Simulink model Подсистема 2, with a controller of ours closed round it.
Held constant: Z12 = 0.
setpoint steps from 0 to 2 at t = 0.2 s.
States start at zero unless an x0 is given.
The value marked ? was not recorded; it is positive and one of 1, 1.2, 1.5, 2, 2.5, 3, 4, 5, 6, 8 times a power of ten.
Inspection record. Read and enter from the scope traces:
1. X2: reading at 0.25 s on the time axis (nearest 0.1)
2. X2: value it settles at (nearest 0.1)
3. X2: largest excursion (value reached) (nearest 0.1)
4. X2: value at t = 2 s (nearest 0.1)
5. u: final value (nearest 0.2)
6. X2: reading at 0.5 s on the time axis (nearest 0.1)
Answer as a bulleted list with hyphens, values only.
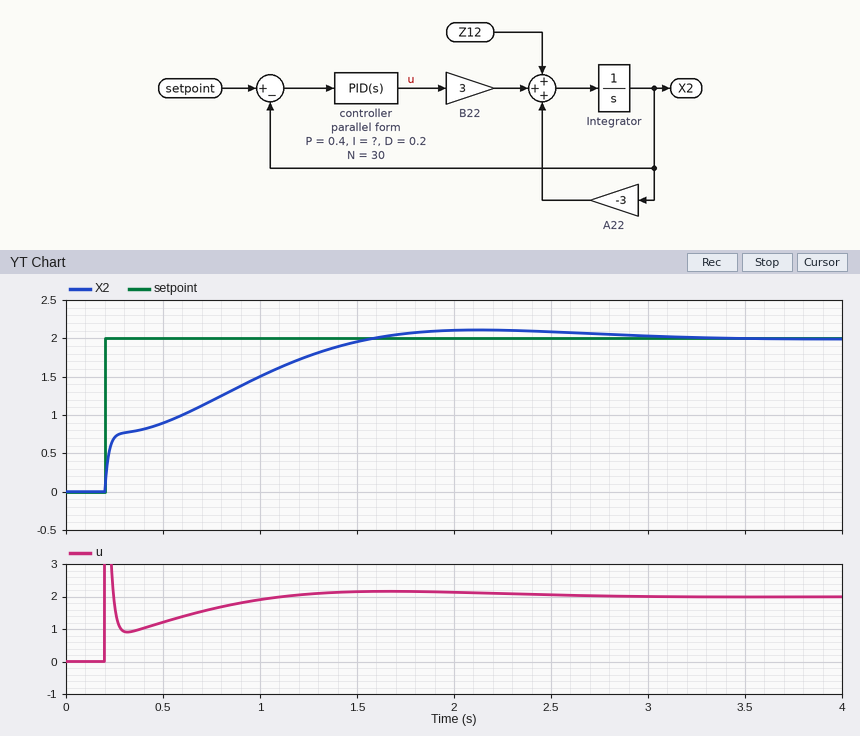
- 0.7
- 2.0
- 2.1
- 2.1
- 2.0
- 0.9
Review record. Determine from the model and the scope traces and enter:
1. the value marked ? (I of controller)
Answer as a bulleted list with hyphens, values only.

- 2.5
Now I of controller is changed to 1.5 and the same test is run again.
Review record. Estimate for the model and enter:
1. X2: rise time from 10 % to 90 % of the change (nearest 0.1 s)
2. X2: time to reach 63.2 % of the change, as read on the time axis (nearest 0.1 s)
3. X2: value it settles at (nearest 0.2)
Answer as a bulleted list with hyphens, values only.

- 1.7 s
- 1.1 s
- 2.0
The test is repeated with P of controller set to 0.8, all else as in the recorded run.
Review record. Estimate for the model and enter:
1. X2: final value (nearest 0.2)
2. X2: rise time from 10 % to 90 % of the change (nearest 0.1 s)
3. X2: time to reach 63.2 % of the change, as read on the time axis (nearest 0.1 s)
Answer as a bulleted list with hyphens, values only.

- 2.0
- 1.1 s
- 0.7 s
